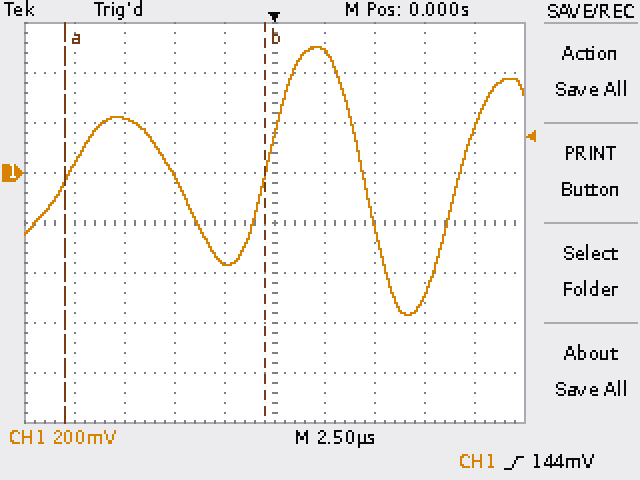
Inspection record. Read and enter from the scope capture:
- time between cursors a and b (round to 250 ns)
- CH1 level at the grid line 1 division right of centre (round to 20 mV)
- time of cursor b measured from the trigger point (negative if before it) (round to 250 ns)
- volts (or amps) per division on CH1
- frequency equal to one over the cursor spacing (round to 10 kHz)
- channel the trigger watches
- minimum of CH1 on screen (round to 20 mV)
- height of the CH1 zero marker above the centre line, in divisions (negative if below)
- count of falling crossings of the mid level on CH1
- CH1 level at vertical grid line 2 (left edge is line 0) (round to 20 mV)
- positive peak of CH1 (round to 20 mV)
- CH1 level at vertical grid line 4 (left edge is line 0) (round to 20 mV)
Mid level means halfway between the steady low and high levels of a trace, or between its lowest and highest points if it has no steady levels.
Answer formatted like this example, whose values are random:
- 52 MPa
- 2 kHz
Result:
- 10.00 µs
- 480 mV
- -500 ns
- 200 mV
- 100 kHz
- CH1
- -560 mV
- +1.0 div
- 2
- 220 mV
- 500 mV
- -360 mV
